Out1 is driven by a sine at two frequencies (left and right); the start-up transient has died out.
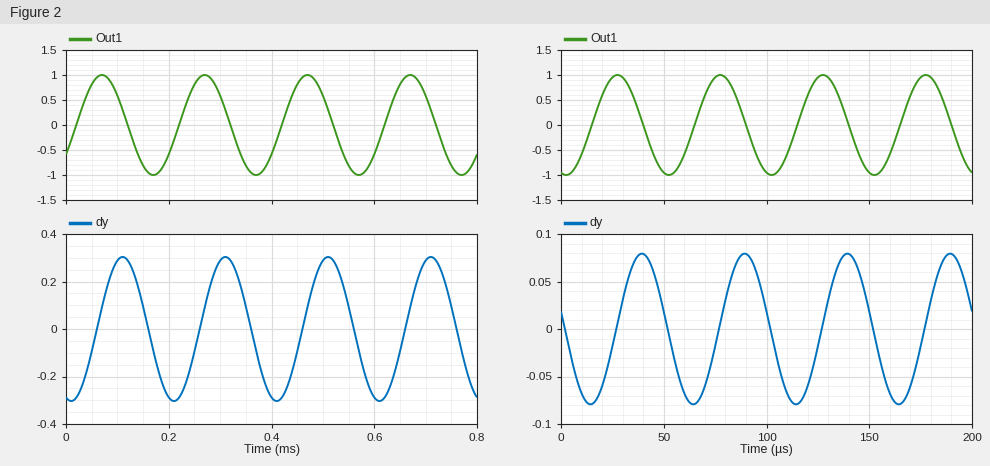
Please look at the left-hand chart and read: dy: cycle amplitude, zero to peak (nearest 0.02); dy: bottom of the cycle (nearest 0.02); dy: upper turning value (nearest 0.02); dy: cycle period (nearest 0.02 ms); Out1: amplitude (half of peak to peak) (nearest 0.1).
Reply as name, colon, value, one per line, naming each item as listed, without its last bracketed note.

dy: cycle amplitude, zero to peak: 0.30
dy: bottom of the cycle: -0.30
dy: upper turning value: 0.30
dy: cycle period: 0.20 ms
Out1: amplitude (half of peak to peak): 1.0
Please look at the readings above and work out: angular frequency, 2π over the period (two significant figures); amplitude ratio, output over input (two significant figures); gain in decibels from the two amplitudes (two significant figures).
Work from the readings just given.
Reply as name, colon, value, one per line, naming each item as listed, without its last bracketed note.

angular frequency, 2π over the period: 31 rad/ms
amplitude ratio, output over input: 0.30
gain in decibels from the two amplitudes: -10 dB
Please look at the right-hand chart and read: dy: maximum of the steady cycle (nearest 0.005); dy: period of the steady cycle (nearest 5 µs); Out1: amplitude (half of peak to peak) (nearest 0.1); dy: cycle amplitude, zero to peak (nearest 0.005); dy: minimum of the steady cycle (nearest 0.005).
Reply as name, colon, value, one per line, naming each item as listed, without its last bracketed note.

dy: maximum of the steady cycle: 0.080
dy: period of the steady cycle: 50 µs
Out1: amplitude (half of peak to peak): 1.0
dy: cycle amplitude, zero to peak: 0.080
dy: minimum of the steady cycle: -0.080
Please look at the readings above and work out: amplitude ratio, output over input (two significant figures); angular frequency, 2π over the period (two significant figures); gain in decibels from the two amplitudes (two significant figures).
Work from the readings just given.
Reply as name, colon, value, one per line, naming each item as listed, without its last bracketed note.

amplitude ratio, output over input: 0.080
angular frequency, 2π over the period: 0.13 rad/µs
gain in decibels from the two amplitudes: -22 dB
